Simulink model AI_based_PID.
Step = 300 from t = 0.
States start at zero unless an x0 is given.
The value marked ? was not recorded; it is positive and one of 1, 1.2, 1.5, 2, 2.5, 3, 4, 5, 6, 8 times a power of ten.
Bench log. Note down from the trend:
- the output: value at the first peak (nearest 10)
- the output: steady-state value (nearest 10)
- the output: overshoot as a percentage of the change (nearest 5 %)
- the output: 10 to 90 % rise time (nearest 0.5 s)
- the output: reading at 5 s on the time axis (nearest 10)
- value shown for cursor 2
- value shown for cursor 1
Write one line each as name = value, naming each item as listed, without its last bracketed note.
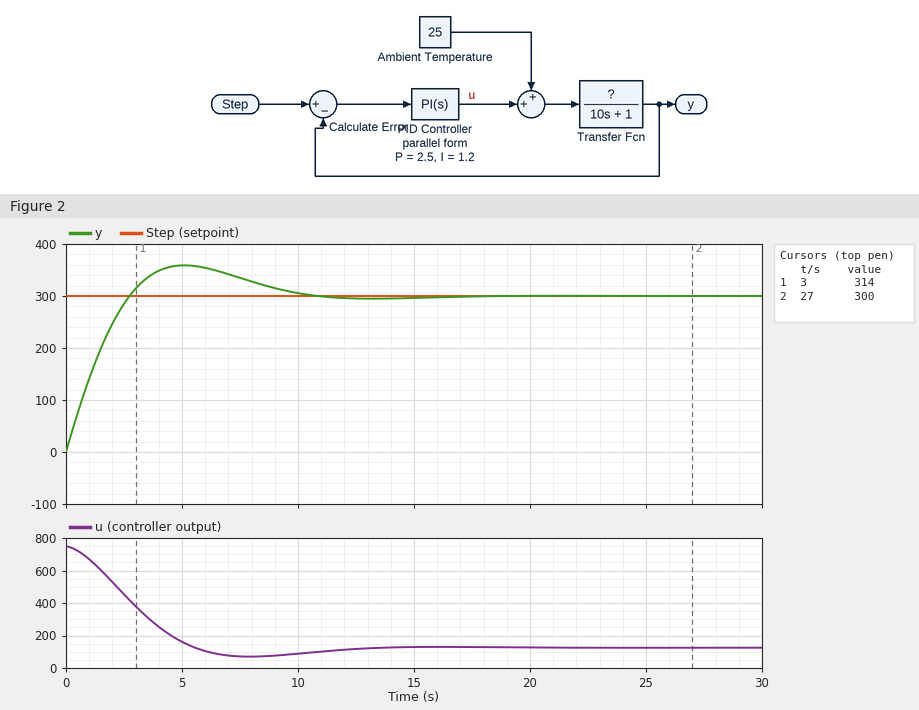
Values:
the output: value at the first peak = 360
the output: steady-state value = 300
the output: overshoot as a percentage of the change = 20 %
the output: 10 to 90 % rise time = 2.0 s
the output: reading at 5 s on the time axis = 360
value shown for cursor 2 = 300
value shown for cursor 1 = 314
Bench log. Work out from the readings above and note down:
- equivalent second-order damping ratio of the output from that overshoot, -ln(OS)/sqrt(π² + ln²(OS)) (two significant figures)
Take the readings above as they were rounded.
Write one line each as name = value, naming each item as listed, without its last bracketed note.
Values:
equivalent second-order damping ratio of the output from that overshoot, -ln(OS)/sqrt(π² + ln²(OS)) = 0.46
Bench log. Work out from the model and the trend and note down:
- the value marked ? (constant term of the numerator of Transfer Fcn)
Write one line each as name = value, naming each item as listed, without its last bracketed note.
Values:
the value marked ? = 2
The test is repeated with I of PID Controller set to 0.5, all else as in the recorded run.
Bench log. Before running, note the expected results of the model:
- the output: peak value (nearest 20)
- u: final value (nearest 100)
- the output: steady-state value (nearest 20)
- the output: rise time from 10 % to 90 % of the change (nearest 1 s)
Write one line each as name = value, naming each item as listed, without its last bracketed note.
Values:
the output: peak value = 320
u: final value = 100
the output: steady-state value = 300
the output: rise time from 10 % to 90 % of the change = 3 s
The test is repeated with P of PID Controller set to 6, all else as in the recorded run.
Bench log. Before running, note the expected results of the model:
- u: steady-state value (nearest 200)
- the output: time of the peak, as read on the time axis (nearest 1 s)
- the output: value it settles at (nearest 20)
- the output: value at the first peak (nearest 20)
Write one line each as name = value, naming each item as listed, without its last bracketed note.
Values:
u: steady-state value = 200
the output: time of the peak, as read on the time axis = 4 s
the output: value it settles at = 300
the output: value at the first peak = 320
